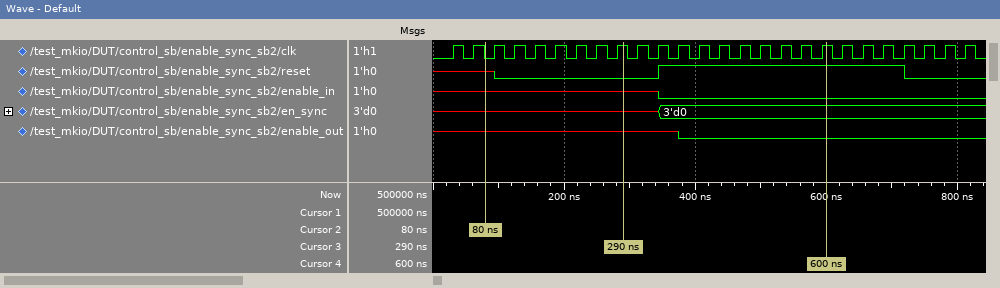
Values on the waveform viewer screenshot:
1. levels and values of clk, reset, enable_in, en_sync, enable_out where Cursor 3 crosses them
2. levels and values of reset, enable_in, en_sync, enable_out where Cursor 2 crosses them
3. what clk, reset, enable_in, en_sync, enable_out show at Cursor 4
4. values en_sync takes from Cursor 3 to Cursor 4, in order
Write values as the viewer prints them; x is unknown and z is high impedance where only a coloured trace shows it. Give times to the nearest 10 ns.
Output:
clk=1, reset=0, enable_in=x, en_sync=x, enable_out=x
reset=x, enable_in=x, en_sync=x, enable_out=x
clk=1, reset=1, enable_in=0, en_sync=3'd0, enable_out=0
x, 3'd0
